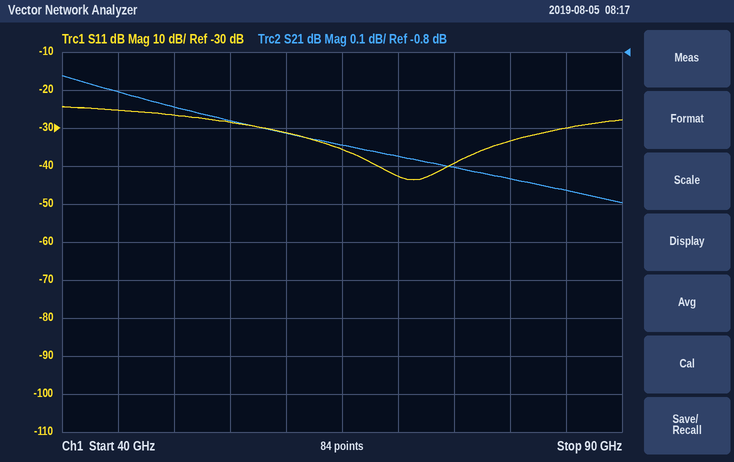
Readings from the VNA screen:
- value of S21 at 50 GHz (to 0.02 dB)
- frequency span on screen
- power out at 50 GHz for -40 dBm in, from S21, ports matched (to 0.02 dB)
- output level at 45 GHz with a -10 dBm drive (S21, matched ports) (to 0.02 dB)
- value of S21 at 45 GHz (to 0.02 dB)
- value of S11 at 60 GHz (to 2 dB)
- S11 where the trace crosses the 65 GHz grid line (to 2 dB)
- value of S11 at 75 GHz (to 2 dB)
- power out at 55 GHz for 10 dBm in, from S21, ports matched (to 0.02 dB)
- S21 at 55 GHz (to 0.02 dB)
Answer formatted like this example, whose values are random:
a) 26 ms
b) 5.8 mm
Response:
a) -0.94 dB
b) 50 GHz
c) -40.94 dBm
d) -10.90 dBm
e) -0.90 dB
f) -32 dB
g) -36 dB
h) -40 dB
i) 9.02 dBm
j) -0.98 dB
